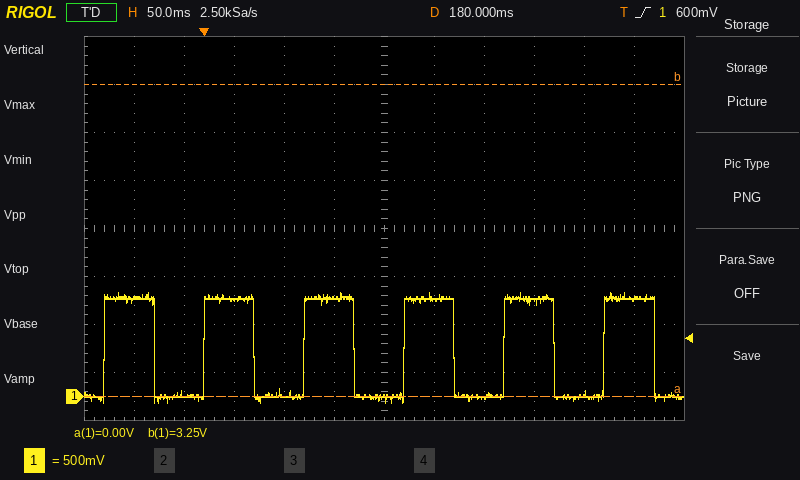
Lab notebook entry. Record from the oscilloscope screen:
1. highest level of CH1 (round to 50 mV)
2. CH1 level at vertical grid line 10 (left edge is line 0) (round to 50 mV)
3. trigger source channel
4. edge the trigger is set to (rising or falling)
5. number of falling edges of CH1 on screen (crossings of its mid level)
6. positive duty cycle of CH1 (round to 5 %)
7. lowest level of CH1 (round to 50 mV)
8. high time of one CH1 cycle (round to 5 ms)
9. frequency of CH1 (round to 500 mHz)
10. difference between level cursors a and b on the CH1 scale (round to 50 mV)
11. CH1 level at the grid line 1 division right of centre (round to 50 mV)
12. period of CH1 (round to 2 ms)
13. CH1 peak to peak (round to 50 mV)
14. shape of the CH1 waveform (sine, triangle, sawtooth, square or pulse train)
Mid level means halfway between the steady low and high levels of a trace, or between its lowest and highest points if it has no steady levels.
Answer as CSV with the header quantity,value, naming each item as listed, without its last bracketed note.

quantity,value
highest level of CH1,1.10 V
CH1 level at vertical grid line 10 (left edge is line 0),50 mV
trigger source channel,CH1
edge the trigger is set to,rising
number of falling edges of CH1 on screen,6
positive duty cycle of CH1,50 %
lowest level of CH1,-50 mV
high time of one CH1 cycle,50 ms
frequency of CH1,10.0 Hz
difference between level cursors a and b on the CH1 scale,3.25 V
CH1 level at the grid line 1 division right of centre,1.00 V
period of CH1,100 ms
CH1 peak to peak,1.15 V
shape of the CH1 waveform,square
